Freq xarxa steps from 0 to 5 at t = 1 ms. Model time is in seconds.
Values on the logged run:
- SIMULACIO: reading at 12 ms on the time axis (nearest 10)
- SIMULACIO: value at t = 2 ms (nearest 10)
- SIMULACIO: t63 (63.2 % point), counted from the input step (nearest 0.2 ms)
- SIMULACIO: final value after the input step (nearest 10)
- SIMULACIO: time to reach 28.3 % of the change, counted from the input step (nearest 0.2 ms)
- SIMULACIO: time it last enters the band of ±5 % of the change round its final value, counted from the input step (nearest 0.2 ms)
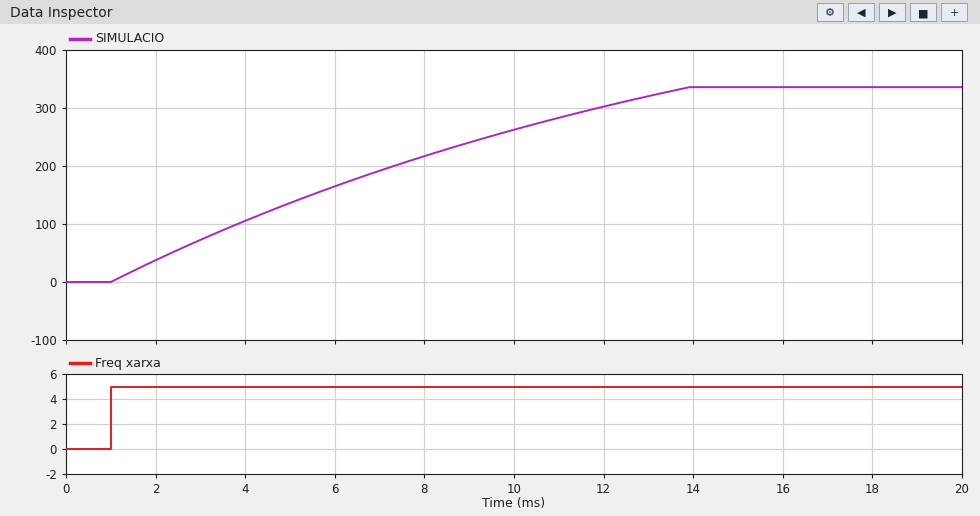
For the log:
300
40
6.8 ms
340
2.6 ms
12.0 ms
